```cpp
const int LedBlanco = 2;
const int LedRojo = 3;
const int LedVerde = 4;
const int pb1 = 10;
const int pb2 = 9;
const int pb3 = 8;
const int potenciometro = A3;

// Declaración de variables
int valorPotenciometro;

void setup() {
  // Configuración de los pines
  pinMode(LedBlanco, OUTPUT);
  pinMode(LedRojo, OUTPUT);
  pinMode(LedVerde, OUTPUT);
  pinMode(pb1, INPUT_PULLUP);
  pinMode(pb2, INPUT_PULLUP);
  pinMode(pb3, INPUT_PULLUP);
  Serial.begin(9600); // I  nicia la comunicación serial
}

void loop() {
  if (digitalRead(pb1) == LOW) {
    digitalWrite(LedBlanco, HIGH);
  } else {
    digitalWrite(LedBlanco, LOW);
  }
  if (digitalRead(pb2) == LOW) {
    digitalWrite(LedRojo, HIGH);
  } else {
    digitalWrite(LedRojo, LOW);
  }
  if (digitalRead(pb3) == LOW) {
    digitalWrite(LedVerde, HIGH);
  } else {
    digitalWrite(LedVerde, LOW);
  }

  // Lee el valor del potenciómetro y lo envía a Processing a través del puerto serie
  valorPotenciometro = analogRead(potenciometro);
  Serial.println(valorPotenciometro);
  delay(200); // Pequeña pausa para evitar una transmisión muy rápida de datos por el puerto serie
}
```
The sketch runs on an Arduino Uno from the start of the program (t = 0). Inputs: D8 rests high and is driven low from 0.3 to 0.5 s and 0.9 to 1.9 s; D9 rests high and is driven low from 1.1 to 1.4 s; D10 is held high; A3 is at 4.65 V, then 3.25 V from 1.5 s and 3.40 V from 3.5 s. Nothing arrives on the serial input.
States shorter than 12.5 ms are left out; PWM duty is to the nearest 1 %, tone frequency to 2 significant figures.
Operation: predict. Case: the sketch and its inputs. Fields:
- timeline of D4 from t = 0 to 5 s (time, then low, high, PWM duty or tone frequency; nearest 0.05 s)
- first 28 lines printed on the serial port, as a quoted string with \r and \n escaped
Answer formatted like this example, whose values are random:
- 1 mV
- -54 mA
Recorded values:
- 0 s low; 0.4 s high; 0.6 s low; 1 s high; 2 s low
- "952\r\n952\r\n952\r\n952\r\n952\r\n952\r\n952\r\n952\r\n665\r\n665\r\n665\r\n665\r\n665\r\n665\r\n665\r\n665\r\n665\r\n665\r\n696\r\n696\r\n696\r\n696\r\n696\r\n696\r\n696\r\n696\r\n696\r\n696\r\n"
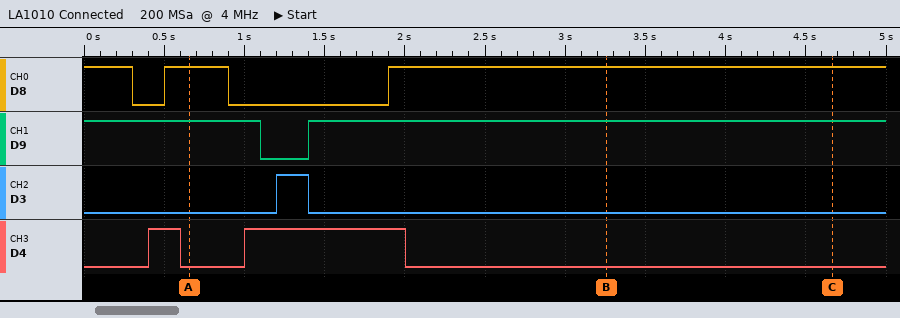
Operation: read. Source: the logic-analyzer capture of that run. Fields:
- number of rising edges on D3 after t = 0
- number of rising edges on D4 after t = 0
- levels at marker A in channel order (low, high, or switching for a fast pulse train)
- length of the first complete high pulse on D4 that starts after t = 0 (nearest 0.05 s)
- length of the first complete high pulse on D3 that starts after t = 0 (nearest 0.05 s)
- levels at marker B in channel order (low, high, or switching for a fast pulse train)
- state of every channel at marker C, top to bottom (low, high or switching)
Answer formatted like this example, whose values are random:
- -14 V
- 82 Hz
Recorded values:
- 1
- 2
- D8 high, D9 high, D3 low, D4 low
- 0.20 s
- 0.20 s
- D8 high, D9 high, D3 low, D4 low
- D8 high, D9 high, D3 low, D4 low
